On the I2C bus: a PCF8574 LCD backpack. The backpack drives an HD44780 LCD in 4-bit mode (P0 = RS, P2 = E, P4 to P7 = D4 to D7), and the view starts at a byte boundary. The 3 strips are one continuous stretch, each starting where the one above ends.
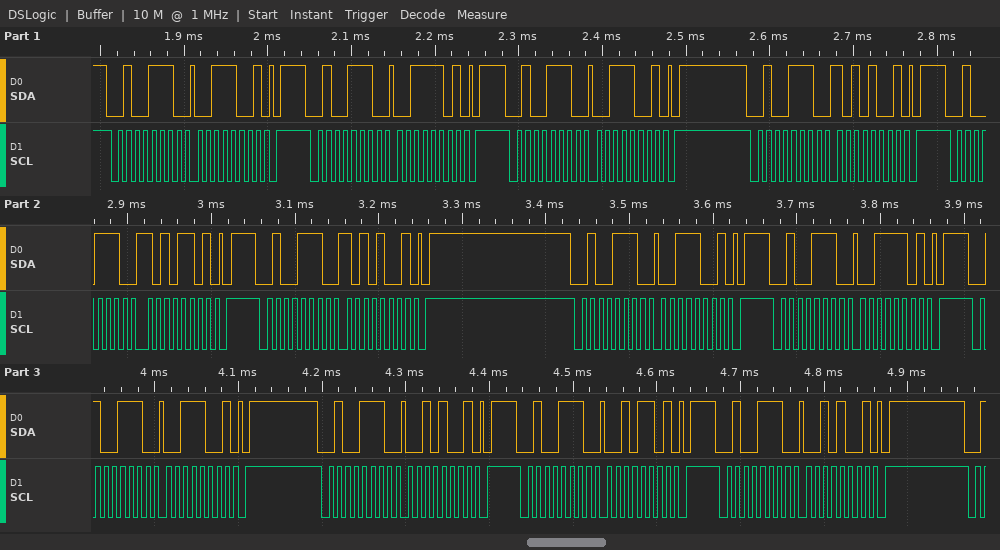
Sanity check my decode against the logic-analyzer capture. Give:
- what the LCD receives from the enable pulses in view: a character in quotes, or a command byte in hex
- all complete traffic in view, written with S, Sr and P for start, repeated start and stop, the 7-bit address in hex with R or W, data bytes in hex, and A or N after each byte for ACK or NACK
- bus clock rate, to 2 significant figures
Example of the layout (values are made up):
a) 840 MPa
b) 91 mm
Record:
a) ':' '2'
b) S 27W A 39 A P S 27W A 3D A P S 27W A 39 A P S 27W A A9 A P S 27W A AD A P S 27W A A9 A P S 27W A 39 A P S 27W A 3D A P S 27W A 39 A P S 27W A 29 A P S 27W A 2D A P S 27W A 29 A P
c) 100 kHz
